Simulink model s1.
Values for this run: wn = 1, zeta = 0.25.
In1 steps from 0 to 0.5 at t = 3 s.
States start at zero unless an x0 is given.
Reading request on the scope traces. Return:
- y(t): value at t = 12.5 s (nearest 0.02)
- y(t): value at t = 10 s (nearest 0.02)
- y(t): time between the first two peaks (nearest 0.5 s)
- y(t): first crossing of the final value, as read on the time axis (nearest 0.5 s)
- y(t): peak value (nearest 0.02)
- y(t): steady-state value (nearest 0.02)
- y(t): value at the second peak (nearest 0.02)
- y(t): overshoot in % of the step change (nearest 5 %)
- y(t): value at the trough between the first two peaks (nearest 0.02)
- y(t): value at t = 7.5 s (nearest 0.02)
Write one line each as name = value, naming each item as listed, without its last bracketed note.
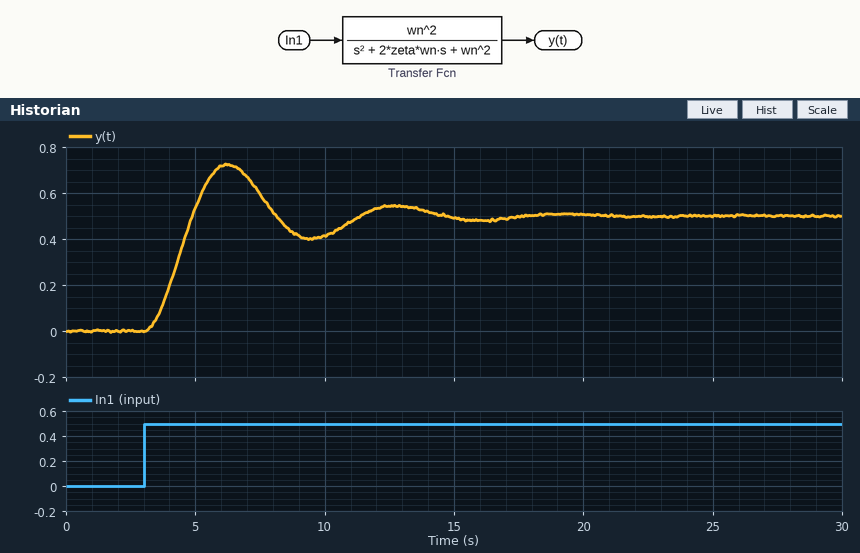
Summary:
y(t): value at t = 12.5 s = 0.54
y(t): value at t = 10 s = 0.42
y(t): time between the first two peaks = 6.5 s
y(t): first crossing of the final value, as read on the time axis = 5.0 s
y(t): peak value = 0.72
y(t): steady-state value = 0.50
y(t): value at the second peak = 0.54
y(t): overshoot in % of the step change = 45 %
y(t): value at the trough between the first two peaks = 0.40
y(t): value at t = 7.5 s = 0.60
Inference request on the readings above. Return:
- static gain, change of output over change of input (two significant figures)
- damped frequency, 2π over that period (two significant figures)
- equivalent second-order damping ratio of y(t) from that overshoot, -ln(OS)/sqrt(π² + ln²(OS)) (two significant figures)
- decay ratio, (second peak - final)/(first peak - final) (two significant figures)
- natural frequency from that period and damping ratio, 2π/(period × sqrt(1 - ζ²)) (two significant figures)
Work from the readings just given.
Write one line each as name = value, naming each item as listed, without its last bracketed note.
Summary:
static gain, change of output over change of input = 1.0
damped frequency, 2π over that period = 0.97 rad/s
equivalent second-order damping ratio of y(t) from that overshoot, -ln(OS)/sqrt(π² + ln²(OS)) = 0.25
decay ratio, (second peak - final)/(first peak - final) = 0.18
natural frequency from that period and damping ratio, 2π/(period × sqrt(1 - ζ²)) = 1.00 rad/s
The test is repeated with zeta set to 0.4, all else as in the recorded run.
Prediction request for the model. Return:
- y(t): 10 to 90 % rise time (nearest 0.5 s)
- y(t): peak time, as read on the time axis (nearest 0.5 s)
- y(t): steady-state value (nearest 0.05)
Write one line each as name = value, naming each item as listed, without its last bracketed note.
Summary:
y(t): 10 to 90 % rise time = 1.5 s
y(t): peak time, as read on the time axis = 6.5 s
y(t): steady-state value = 0.50
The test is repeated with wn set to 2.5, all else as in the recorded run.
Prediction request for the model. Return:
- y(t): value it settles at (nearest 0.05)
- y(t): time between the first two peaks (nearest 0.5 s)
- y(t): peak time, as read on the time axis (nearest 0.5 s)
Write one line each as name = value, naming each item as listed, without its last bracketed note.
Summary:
y(t): value it settles at = 0.50
y(t): time between the first two peaks = 2.5 s
y(t): peak time, as read on the time axis = 4.5 s
